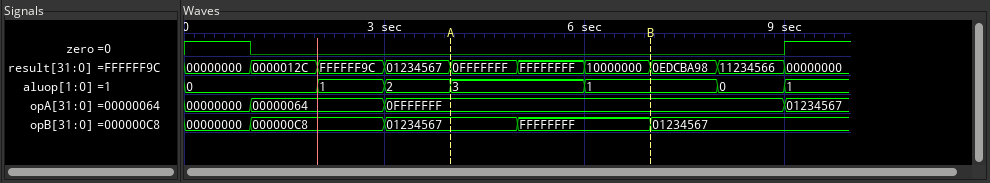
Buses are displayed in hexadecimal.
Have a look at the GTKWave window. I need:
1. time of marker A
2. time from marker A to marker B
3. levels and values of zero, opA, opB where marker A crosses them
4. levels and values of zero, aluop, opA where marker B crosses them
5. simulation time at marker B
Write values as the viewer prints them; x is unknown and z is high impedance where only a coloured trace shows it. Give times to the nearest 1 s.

4 s
3 s
zero=0, opA=0FFFFFFF, opB=01234567
zero=0, aluop=1, opA=0FFFFFFF
7 s
